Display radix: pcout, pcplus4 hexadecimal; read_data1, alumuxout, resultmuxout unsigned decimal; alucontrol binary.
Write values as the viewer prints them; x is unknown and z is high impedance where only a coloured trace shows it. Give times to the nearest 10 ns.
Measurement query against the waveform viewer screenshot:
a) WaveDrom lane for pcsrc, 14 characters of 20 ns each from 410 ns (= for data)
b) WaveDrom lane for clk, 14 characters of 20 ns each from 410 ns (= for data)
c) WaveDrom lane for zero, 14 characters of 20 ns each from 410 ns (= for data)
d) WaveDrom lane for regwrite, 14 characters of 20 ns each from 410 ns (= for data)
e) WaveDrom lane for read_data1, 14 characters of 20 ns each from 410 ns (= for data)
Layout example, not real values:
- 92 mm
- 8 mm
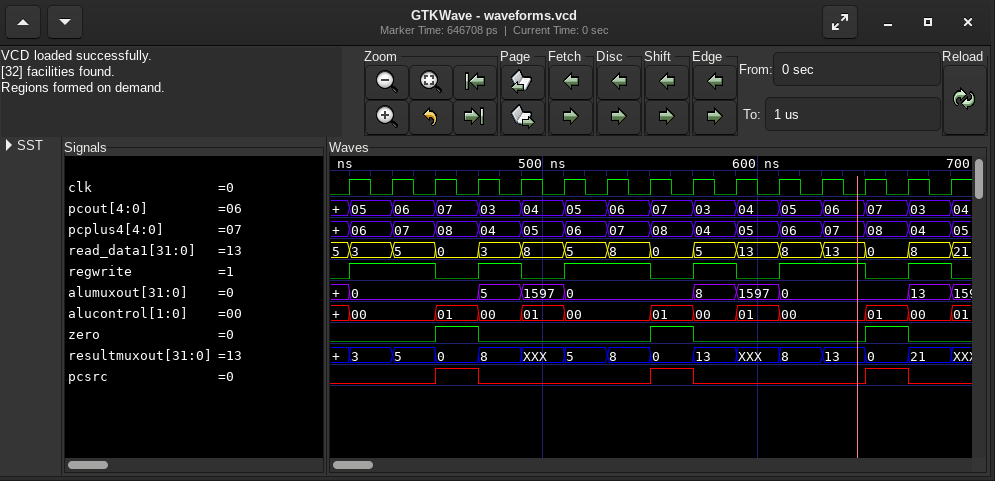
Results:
- {name: 'pcsrc', wave: '0.10...10...10'}
- {name: 'clk', wave: 'p.............'}
- {name: 'zero', wave: '0.10...10...10'}
- {name: 'regwrite', wave: '1.0101.0101.01'}
- {name: 'read_data1', wave: '==============', data: '3 5 0 3 8 5 8 0 5 13 8 13 0 8'}
